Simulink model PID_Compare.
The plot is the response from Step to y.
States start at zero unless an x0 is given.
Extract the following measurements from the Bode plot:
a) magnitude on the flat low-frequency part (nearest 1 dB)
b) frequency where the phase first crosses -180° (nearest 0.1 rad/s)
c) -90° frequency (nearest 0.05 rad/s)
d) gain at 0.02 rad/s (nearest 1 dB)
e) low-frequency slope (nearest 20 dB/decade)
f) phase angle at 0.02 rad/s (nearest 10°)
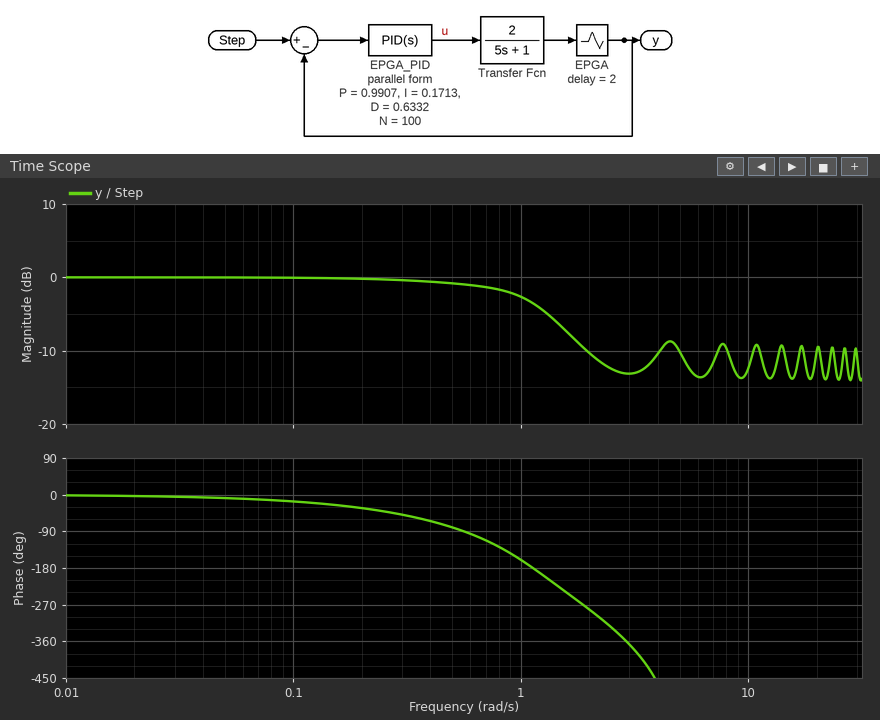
0 dB
1.1 rad/s
0.55 rad/s
0 dB
0 dB/decade
0°
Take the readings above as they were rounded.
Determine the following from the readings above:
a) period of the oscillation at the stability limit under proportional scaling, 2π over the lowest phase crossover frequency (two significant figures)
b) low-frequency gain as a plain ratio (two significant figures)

5.7 s
1.0
